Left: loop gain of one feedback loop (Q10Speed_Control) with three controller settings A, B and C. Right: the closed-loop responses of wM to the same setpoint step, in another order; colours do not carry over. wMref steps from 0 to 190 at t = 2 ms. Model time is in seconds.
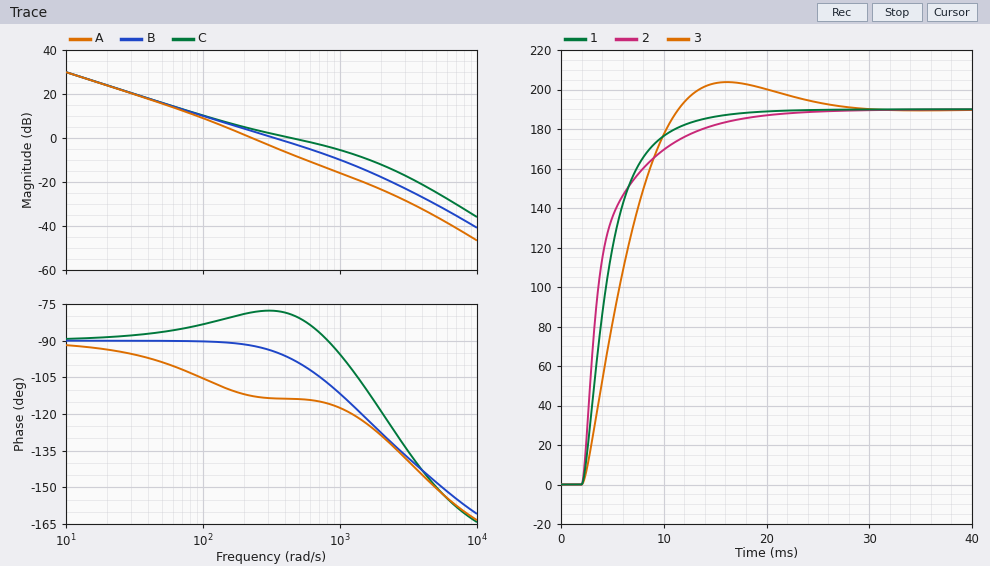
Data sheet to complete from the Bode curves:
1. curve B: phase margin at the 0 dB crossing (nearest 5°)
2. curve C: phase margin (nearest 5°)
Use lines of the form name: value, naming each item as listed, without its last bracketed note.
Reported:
curve B: phase margin at the 0 dB crossing: 85°
curve C: phase margin: 100°
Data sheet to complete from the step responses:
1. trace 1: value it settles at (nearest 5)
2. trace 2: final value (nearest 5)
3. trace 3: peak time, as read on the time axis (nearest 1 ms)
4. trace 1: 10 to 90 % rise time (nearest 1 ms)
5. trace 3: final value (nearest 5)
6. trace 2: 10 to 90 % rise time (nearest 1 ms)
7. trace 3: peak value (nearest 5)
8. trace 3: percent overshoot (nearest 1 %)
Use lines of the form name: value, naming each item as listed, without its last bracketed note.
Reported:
trace 1: value it settles at: 190
trace 2: final value: 190
trace 3: peak time, as read on the time axis: 16 ms
trace 1: 10 to 90 % rise time: 6 ms
trace 3: final value: 190
trace 2: 10 to 90 % rise time: 8 ms
trace 3: peak value: 205
trace 3: percent overshoot: 7 %
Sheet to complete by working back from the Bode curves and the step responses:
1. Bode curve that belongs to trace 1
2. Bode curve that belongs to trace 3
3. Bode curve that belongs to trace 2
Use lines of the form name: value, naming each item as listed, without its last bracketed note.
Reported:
Bode curve that belongs to trace 1: B
Bode curve that belongs to trace 3: A
Bode curve that belongs to trace 2: C
